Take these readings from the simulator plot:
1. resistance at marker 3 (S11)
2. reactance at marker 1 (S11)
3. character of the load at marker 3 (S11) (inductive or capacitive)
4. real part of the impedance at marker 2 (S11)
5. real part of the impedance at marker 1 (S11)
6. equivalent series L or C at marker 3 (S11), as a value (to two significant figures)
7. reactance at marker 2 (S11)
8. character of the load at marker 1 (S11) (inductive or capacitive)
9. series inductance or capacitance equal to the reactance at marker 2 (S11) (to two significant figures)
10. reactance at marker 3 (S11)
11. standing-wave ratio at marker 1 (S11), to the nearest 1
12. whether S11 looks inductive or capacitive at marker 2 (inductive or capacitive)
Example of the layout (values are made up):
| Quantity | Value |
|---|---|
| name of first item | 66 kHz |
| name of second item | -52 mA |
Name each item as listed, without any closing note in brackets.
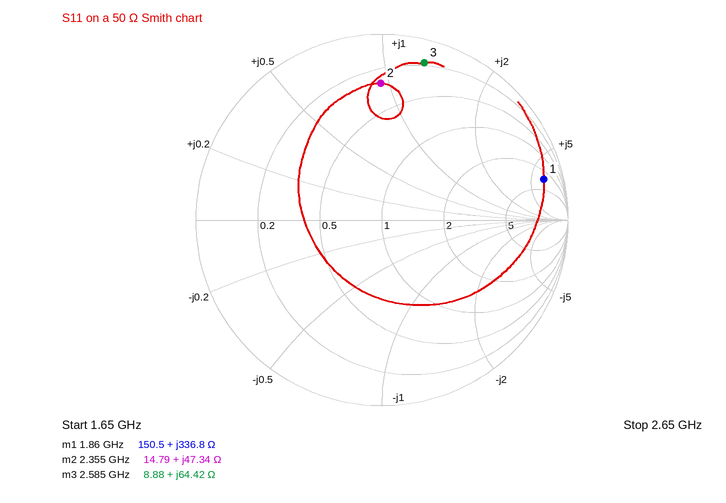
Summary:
| Quantity | Value |
|---|---|
| resistance at marker 3 | 8.88 Ω |
| reactance at marker 1 | +336.8 Ω |
| character of the load at marker 3 (S11) | inductive |
| real part of the impedance at marker 2 | 14.79 Ω |
| real part of the impedance at marker 1 | 150.5 Ω |
| equivalent series L or C at marker 3 (S11), as a value | 4.0 nH |
| reactance at marker 2 | +47.34 Ω |
| character of the load at marker 1 (S11) | inductive |
| series inductance or capacitance equal to the reactance at marker 2 (S11) | 3.2 nH |
| reactance at marker 3 | +64.42 Ω |
| standing-wave ratio at marker 1 (S11), to the nearest 1 | 18 |
| whether S11 looks inductive or capacitive at marker 2 | inductive |
